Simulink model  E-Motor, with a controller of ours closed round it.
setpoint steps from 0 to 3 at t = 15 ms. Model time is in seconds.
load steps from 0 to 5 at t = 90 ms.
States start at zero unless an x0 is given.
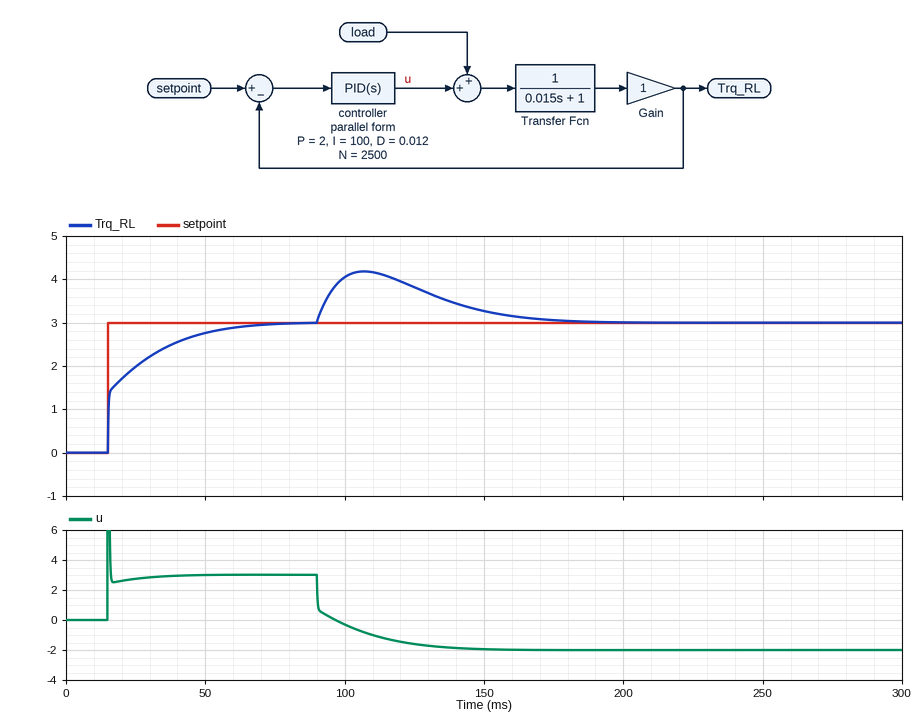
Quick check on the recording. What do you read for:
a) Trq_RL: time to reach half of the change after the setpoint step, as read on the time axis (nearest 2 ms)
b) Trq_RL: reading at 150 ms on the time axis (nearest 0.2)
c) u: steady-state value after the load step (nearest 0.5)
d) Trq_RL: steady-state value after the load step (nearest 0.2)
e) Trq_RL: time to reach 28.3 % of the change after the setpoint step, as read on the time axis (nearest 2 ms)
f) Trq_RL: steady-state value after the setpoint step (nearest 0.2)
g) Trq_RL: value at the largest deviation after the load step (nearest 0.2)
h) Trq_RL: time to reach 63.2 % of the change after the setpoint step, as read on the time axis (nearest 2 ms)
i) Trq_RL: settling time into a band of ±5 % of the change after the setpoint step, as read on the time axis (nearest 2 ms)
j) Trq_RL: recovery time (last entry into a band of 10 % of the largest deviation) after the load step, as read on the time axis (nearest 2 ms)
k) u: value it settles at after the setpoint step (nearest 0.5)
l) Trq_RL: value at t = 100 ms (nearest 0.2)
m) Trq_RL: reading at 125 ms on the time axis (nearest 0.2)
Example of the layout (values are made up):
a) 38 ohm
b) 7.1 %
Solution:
a) 16 ms
b) 3.2
c) -2.0
d) 3.0
e) 16 ms
f) 3.0
g) 4.2
h) 24 ms
i) 56 ms
j) 164 ms
k) 3.0
l) 4.0
m) 3.8
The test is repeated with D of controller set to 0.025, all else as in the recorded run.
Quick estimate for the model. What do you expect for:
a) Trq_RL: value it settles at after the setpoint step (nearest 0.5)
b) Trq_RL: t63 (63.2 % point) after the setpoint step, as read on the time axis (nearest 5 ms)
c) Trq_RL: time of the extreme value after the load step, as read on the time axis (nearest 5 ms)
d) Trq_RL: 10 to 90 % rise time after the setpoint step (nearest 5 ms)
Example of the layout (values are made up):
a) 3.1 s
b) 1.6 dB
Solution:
a) 3.0
b) 15 ms
c) 110 ms
d) 40 ms
